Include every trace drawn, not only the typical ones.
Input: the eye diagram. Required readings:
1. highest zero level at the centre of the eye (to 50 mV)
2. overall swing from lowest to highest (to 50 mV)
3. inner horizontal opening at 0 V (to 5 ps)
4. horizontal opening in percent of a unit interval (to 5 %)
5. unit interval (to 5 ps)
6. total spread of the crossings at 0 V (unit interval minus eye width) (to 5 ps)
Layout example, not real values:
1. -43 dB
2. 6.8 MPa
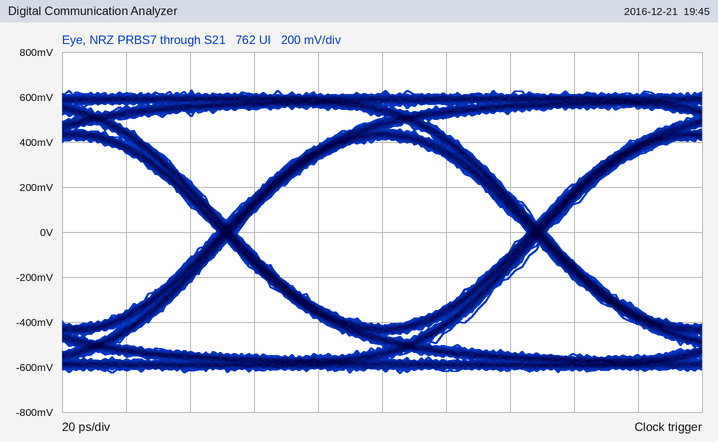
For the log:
1. -400 mV
2. 1.25 V
3. 90 ps
4. 95 %
5. 95 ps
6. 5 ps
